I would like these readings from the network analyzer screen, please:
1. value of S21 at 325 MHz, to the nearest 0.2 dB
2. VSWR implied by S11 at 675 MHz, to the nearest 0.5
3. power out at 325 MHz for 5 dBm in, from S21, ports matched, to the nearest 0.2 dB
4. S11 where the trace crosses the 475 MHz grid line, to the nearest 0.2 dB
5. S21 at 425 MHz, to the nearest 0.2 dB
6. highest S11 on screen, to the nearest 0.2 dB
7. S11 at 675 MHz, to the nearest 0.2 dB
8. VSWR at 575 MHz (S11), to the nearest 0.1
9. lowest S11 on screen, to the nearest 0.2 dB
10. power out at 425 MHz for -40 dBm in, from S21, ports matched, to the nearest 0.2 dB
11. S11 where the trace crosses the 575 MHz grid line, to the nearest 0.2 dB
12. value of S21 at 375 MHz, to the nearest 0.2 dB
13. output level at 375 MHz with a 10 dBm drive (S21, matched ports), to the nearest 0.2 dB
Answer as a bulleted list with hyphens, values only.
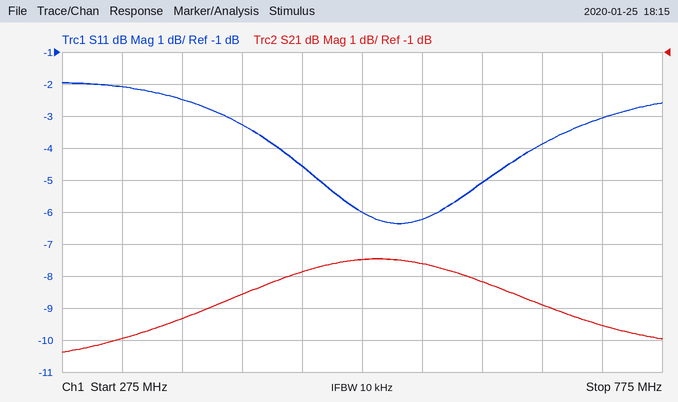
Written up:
- -10.0 dB
- 4.5
- -5.0 dBm
- -4.6 dB
- -8.6 dB
- -2.0 dB
- -3.8 dB
- 2.9
- -6.4 dB
- -48.6 dBm
- -6.2 dB
- -9.4 dB
- 0.6 dBm
